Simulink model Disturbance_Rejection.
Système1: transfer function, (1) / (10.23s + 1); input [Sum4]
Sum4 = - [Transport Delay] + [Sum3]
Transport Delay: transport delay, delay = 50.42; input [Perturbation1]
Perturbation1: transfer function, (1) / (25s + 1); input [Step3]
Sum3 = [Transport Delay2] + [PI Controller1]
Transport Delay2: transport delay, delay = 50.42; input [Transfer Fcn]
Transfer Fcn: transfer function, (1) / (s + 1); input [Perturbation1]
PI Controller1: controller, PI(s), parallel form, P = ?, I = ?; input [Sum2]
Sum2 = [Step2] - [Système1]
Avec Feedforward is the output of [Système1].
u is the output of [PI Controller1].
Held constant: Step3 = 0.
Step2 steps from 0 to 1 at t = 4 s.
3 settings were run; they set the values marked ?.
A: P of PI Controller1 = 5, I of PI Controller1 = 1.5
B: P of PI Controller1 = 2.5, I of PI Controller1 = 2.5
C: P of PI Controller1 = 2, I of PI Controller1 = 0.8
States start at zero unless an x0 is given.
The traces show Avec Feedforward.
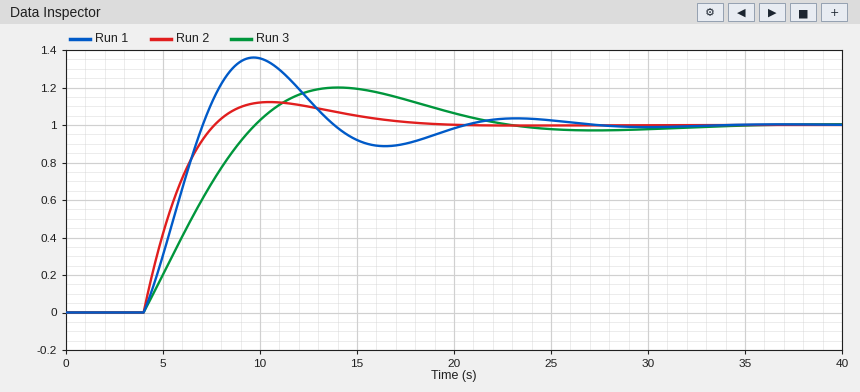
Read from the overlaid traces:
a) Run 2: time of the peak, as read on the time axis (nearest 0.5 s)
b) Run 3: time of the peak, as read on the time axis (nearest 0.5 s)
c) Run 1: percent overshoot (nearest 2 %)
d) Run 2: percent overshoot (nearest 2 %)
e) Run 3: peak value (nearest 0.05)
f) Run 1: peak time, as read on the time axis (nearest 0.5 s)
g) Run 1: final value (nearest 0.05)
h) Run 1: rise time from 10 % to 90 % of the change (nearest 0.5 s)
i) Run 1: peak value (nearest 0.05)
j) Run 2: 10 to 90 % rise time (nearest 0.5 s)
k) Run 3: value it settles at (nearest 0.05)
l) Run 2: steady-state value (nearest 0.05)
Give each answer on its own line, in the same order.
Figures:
10.5 s
14.0 s
36 %
12 %
1.20
9.5 s
1.00
2.5 s
1.35
2.5 s
1.00
1.00
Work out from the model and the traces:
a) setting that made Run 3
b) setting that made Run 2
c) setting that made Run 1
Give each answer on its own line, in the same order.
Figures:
C
A
B
